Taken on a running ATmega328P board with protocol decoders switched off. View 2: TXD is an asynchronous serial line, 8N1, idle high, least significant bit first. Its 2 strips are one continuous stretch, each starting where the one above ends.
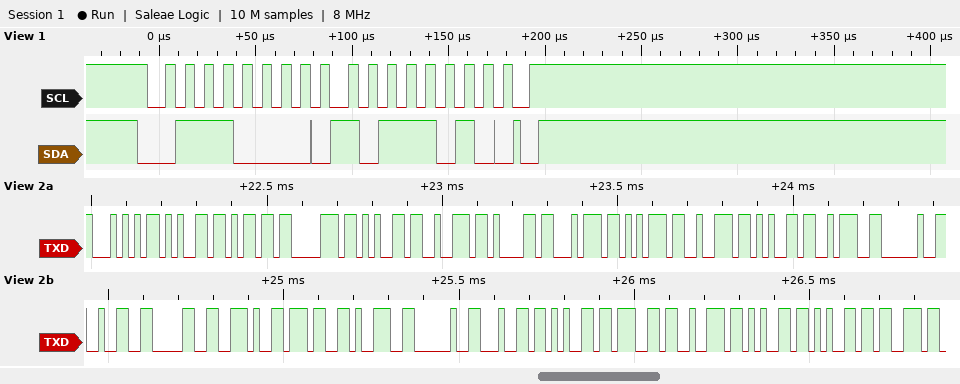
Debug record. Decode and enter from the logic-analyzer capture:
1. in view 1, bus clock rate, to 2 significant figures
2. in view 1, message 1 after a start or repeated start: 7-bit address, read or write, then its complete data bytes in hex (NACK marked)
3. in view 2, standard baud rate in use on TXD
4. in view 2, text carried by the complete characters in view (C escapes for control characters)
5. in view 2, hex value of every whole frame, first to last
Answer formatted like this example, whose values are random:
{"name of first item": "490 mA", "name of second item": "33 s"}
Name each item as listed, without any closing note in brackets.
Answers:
{"in view 1, bus clock rate, to 2 significant figures": "100 kHz", "in view 1, message 1 after a start or repeated start: 7-bit address, read or write, then its complete data bytes in hex": "0x38 write: BA", "in view 2, standard baud rate in use on TXD": "57600 baud", "in view 2, text carried by the complete characters in view": "\"Temperature: 20.79 degrees\"", "in view 2, hex value of every whole frame, first to last": "54 65 6D 70 65 72 61 74 75 72 65 3A 20 32 30 2E 37 39 20 64 65 67 72 65 65 73"}
